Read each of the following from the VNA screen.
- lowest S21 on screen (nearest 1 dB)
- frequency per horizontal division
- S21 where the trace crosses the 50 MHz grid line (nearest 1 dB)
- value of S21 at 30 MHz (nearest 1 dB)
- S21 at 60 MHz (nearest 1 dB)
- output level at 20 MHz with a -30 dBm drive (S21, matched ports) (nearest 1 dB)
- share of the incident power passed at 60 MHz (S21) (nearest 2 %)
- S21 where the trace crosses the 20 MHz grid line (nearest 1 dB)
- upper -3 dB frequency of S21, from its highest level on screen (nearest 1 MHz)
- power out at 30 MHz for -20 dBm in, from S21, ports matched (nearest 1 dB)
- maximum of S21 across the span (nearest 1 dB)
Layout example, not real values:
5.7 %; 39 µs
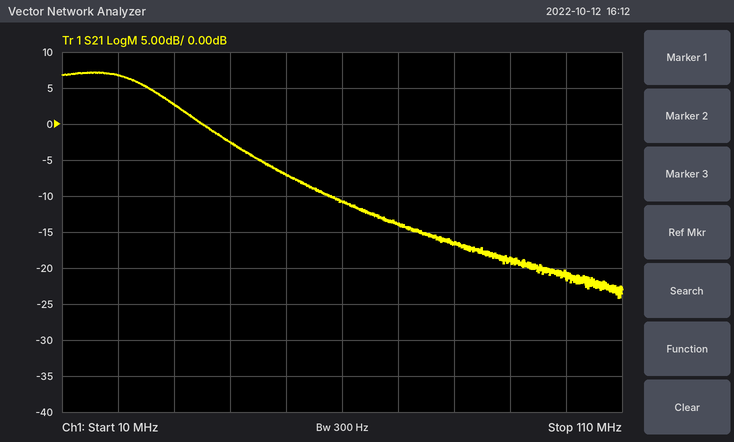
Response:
-24 dB; 10 MHz; -7 dB; 3 dB; -11 dB; -23 dBm; 8 %; 7 dB; 27 MHz; -17 dBm; 7 dB
